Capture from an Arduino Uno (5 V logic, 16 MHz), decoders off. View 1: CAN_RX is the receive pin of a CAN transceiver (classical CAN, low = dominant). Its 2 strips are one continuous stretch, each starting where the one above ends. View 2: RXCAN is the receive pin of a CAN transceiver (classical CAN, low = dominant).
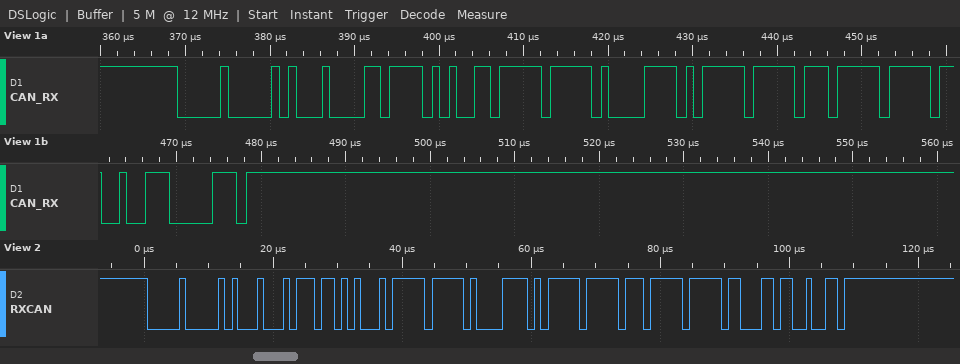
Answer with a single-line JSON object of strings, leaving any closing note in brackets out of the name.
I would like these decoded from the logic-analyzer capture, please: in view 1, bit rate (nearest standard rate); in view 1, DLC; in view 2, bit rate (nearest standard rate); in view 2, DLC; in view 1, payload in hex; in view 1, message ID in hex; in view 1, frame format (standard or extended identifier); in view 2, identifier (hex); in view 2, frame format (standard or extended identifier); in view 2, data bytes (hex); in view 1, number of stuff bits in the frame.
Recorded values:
{"in view 1, bit rate": "1000 kbit/s", "in view 1, DLC": "8", "in view 2, bit rate": "1000 kbit/s", "in view 2, DLC": "8", "in view 1, payload in hex": "6F 53 7F F0 F5 FF F7 FF", "in view 1, message ID in hex": "0x001", "in view 1, frame format": "standard", "in view 2, identifier": "0x001", "in view 2, frame format": "standard", "in view 2, data bytes": "BB 51 7F F0 F5 FF F7 FF", "in view 1, number of stuff bits in the frame": "9"}
